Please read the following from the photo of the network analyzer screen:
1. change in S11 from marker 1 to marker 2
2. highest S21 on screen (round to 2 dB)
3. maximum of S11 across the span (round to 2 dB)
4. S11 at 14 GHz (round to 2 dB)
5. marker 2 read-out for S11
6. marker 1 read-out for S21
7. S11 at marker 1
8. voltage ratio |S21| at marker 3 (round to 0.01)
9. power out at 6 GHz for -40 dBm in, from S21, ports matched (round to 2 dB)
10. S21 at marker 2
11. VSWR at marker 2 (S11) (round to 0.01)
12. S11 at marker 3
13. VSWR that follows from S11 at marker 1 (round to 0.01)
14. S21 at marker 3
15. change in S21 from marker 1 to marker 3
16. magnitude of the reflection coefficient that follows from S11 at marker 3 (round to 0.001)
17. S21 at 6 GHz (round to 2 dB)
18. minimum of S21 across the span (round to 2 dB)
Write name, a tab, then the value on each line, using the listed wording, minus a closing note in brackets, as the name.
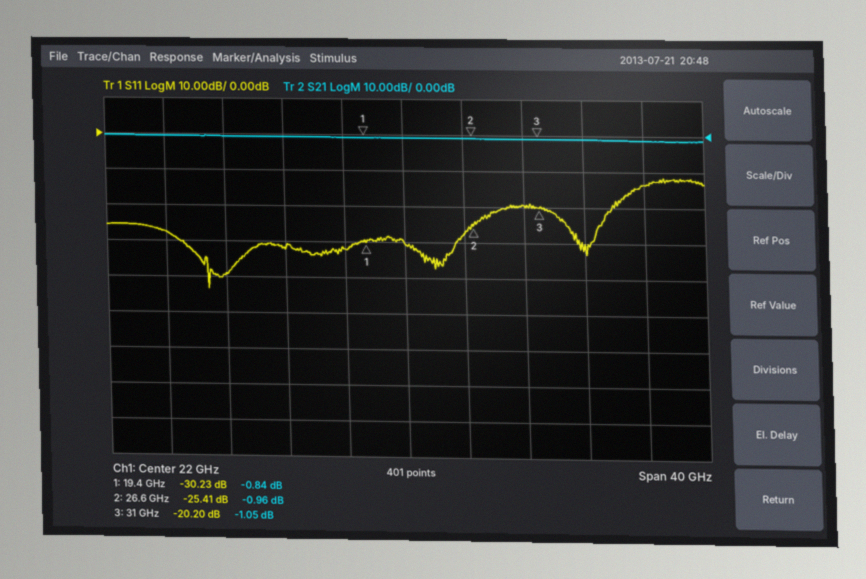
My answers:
change in S11 from marker 1 to marker 2	4.82 dB
highest S21 on screen	0 dB
maximum of S11 across the span	-12 dB
S11 at 14 GHz	-32 dB
marker 2 read-out for S11	-25.41 dB
marker 1 read-out for S21	-0.84 dB
S11 at marker 1	-30.23 dB
voltage ratio |S21| at marker 3	0.89
power out at 6 GHz for -40 dBm in, from S21, ports matched	-40 dBm
S21 at marker 2	-0.96 dB
VSWR at marker 2 (S11)	1.11
S11 at marker 3	-20.20 dB
VSWR that follows from S11 at marker 1	1.06
S21 at marker 3	-1.05 dB
change in S21 from marker 1 to marker 3	-0.21 dB
magnitude of the reflection coefficient that follows from S11 at marker 3	0.098
S21 at 6 GHz	0 dB
minimum of S21 across the span	-2 dB
